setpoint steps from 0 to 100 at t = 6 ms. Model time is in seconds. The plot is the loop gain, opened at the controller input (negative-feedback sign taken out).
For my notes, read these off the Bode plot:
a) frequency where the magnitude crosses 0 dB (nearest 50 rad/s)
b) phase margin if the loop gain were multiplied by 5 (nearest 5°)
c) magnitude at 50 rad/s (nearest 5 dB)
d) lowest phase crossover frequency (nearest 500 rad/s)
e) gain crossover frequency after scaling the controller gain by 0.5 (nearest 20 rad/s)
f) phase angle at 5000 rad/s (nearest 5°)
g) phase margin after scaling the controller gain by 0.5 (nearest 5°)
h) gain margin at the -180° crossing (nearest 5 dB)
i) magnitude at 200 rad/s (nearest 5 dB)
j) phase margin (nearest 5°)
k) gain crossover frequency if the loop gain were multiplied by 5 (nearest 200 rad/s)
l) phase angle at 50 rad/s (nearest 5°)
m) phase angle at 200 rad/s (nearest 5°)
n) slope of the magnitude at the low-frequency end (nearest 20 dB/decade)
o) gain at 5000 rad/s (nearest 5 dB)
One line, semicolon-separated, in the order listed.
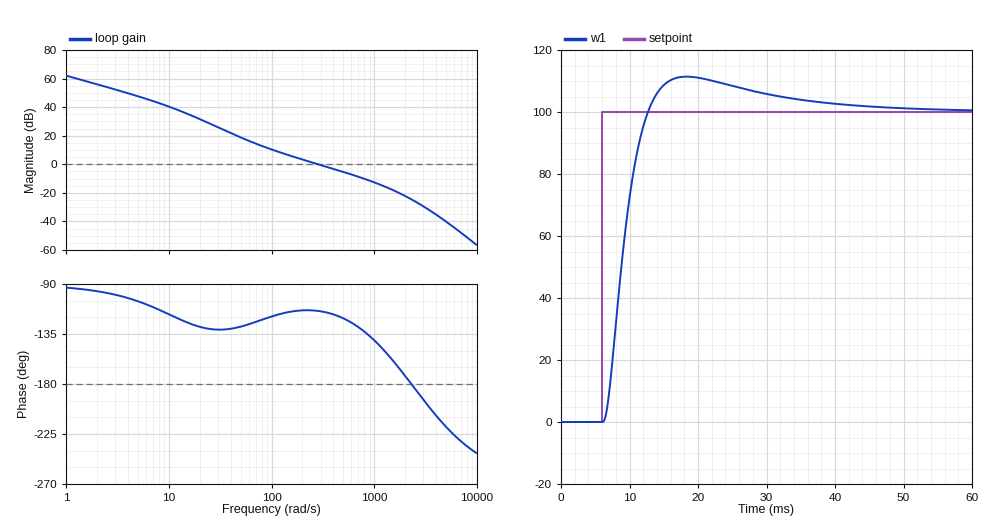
300 rad/s; 35°; 20 dB; 2500 rad/s; 160 rad/s; -220°; 65°; 25 dB; 5 dB; 65°; 1200 rad/s; -130°; -115°; -20 dB/decade; -40 dB
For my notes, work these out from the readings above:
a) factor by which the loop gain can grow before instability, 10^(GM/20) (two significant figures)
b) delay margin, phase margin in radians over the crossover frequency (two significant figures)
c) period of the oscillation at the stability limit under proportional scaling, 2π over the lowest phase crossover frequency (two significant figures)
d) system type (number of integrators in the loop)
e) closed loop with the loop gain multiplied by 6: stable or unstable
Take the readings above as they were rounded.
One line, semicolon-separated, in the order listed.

18; 0.0038 s; 0.0025 s; 1; stable
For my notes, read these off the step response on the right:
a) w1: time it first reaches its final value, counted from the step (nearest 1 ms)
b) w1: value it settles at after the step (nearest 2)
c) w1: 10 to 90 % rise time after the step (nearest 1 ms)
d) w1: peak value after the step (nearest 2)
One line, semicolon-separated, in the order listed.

7 ms; 100; 4 ms; 112
